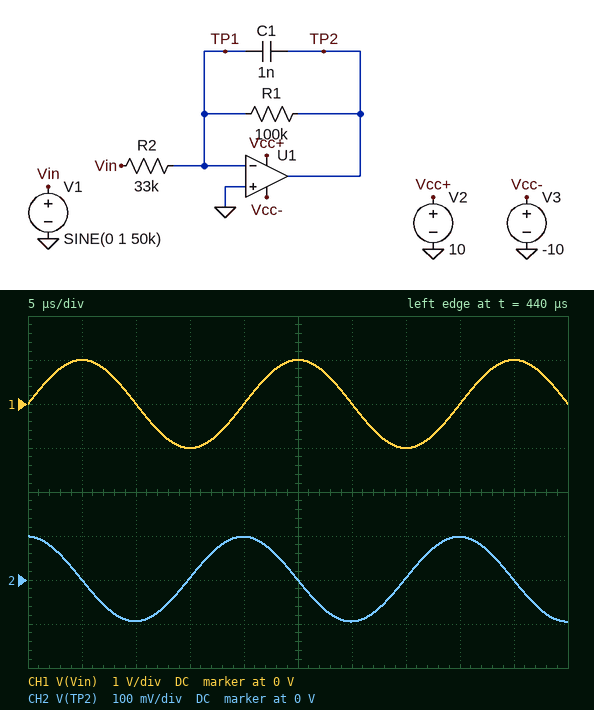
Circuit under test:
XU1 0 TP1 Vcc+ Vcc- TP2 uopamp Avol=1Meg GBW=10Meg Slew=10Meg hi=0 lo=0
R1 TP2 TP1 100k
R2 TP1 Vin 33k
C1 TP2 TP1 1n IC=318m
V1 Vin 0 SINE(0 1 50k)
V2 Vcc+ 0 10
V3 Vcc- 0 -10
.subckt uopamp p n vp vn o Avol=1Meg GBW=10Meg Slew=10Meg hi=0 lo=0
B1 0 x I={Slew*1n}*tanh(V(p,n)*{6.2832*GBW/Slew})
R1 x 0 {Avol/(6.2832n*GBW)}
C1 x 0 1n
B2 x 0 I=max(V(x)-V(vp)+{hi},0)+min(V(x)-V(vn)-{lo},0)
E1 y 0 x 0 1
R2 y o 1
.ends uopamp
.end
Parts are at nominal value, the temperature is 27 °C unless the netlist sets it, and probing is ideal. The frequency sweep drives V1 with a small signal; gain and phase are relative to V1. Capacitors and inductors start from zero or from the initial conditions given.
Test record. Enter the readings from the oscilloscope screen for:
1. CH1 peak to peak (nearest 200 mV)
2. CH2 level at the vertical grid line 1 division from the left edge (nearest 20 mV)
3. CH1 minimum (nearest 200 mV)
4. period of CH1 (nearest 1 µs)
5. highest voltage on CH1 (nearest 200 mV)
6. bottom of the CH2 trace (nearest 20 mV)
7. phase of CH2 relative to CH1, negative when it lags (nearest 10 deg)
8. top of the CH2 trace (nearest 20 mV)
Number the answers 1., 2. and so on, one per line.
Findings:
1. 2.0 V
2. 0 V
3. -1.0 V
4. 20 µs
5. 1.0 V
6. -100 mV
7. 90 deg
8. 100 mV
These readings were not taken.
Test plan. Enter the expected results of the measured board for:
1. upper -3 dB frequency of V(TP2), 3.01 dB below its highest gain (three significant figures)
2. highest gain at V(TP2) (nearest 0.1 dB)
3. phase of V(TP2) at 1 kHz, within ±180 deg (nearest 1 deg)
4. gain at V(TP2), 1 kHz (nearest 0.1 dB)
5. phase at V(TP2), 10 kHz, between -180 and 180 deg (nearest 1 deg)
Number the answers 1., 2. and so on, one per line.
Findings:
1. 1.59 kHz
2. 9.6 dB
3. 148 deg
4. 8.2 dB
5. 99 deg
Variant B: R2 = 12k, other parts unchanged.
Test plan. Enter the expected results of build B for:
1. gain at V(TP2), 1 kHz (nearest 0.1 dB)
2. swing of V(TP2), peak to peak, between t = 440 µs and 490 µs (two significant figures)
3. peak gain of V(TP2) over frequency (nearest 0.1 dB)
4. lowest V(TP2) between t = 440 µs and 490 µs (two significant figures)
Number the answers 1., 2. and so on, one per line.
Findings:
1. 17.0 dB
2. 530 mV
3. 18.4 dB
4. -260 mV
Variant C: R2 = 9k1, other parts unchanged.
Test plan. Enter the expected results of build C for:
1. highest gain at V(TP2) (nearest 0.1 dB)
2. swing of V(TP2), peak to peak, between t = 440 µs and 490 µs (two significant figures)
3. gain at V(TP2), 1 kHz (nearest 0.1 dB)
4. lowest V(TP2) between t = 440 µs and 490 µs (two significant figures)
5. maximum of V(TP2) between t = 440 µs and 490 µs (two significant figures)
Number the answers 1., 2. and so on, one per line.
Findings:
1. 20.8 dB
2. 700 mV
3. 19.4 dB
4. -350 mV
5. 350 mV
